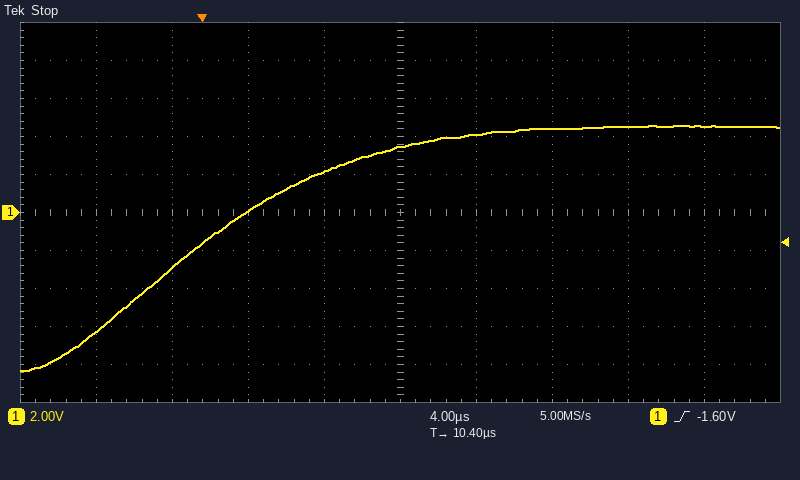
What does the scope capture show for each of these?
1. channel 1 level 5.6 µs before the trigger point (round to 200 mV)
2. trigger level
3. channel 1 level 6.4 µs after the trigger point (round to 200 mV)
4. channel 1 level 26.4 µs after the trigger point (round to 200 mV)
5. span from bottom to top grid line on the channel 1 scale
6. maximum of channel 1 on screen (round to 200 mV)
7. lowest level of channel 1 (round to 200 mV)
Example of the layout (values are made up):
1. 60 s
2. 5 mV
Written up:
1. -6.2 V
2. -1.60 V
3. 2.2 V
4. 4.6 V
5. 20 V
6. 4.6 V
7. -8.4 V
